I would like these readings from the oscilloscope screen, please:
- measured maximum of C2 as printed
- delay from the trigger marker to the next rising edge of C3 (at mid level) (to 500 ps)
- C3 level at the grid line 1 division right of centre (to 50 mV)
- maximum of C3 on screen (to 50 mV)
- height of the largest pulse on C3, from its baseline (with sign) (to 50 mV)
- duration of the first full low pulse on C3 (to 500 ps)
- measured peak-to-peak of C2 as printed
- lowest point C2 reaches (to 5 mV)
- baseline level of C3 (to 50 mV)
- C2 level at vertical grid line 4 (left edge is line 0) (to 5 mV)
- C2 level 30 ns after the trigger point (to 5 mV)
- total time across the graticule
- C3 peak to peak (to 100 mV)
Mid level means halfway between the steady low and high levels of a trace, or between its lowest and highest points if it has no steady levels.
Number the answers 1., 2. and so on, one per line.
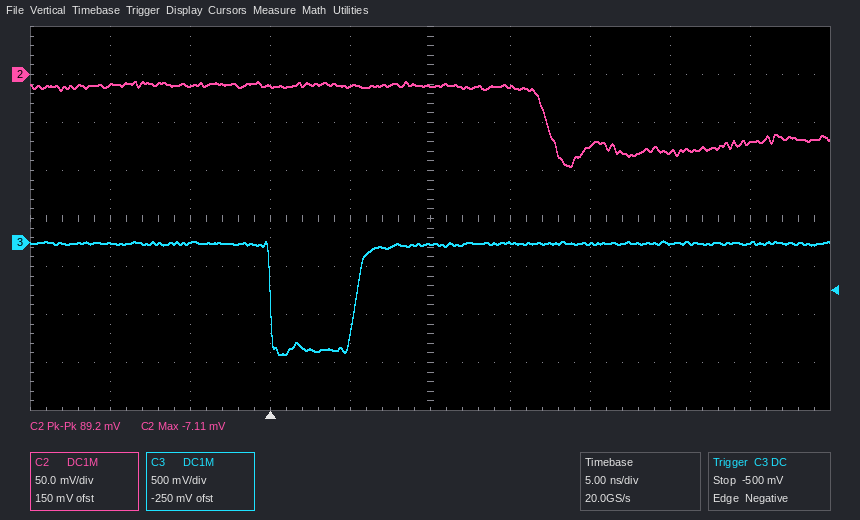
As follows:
1. -7.11 mV
2. 5.5 ns
3. 0 mV
4. 0 mV
5. -1.15 V
6. 5.5 ns
7. 89.2 mV
8. -95 mV
9. 0 mV
10. -10 mV
11. -70 mV
12. 50 ns
13. 1.20 V
